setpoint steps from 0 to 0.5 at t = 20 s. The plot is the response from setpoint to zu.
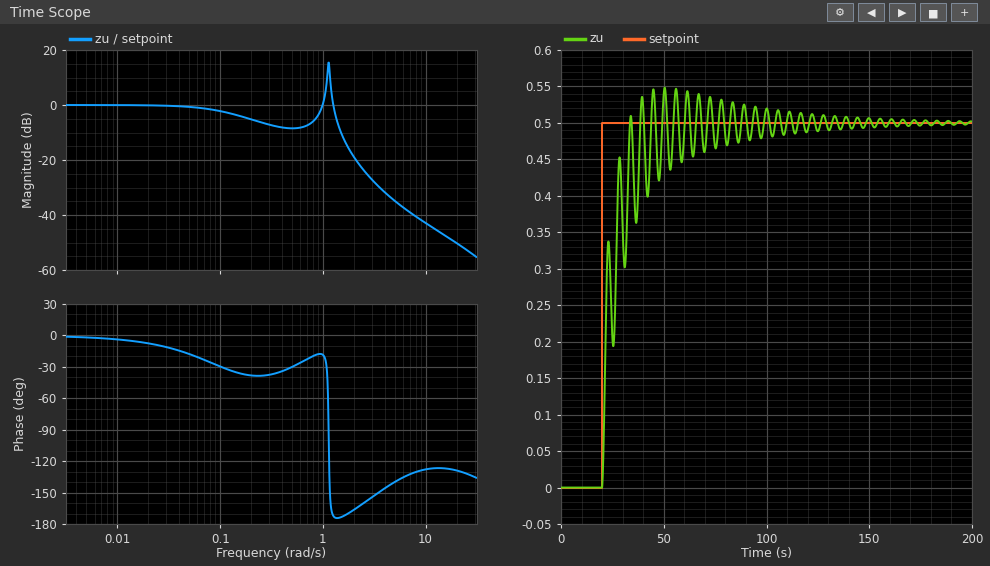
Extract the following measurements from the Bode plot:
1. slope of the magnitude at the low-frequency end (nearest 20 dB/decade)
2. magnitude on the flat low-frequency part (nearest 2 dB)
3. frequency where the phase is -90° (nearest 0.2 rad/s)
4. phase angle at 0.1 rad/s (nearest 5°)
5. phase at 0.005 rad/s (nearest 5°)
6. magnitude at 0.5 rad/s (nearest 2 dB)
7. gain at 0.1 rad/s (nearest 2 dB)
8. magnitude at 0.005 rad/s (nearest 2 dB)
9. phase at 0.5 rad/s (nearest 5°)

0 dB/decade
0 dB
1.2 rad/s
-30°
0°
-8 dB
-2 dB
0 dB
-30°
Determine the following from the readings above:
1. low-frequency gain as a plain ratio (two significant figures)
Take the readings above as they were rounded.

1.0
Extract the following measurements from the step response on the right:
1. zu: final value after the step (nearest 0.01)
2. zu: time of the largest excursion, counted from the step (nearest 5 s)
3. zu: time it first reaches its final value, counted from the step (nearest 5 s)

0.50
30 s
15 s
